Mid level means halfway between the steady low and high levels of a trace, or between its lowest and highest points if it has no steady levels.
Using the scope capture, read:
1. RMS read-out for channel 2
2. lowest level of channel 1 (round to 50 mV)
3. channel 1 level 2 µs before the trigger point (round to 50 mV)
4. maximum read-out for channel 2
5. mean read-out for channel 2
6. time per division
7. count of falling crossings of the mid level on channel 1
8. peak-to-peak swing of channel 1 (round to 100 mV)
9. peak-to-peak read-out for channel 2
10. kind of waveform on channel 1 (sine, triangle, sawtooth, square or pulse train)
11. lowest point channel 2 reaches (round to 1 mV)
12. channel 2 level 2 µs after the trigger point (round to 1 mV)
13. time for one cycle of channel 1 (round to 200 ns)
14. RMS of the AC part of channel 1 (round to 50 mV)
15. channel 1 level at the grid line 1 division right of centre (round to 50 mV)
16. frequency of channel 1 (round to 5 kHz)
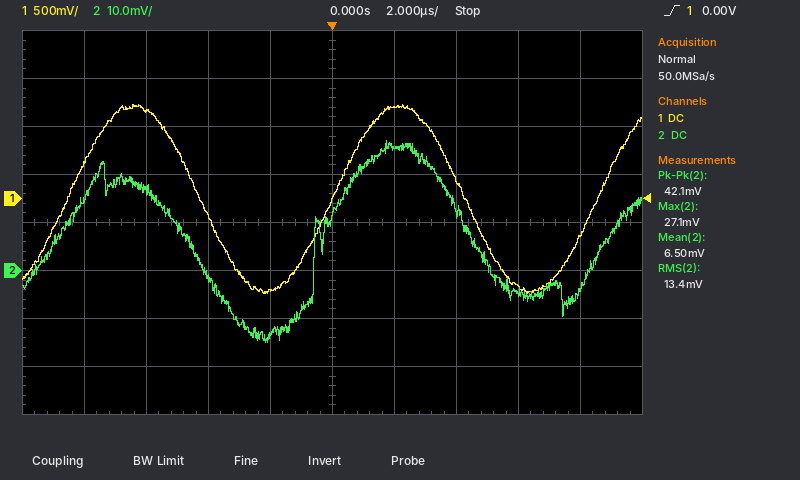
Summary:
13.4 mV
-1.00 V
-950 mV
27.1 mV
6.50 mV
2 µs
2
2.00 V
42.1 mV
sine
-15 mV
26 mV
8.6 µs
700 mV
950 mV
115 kHz
